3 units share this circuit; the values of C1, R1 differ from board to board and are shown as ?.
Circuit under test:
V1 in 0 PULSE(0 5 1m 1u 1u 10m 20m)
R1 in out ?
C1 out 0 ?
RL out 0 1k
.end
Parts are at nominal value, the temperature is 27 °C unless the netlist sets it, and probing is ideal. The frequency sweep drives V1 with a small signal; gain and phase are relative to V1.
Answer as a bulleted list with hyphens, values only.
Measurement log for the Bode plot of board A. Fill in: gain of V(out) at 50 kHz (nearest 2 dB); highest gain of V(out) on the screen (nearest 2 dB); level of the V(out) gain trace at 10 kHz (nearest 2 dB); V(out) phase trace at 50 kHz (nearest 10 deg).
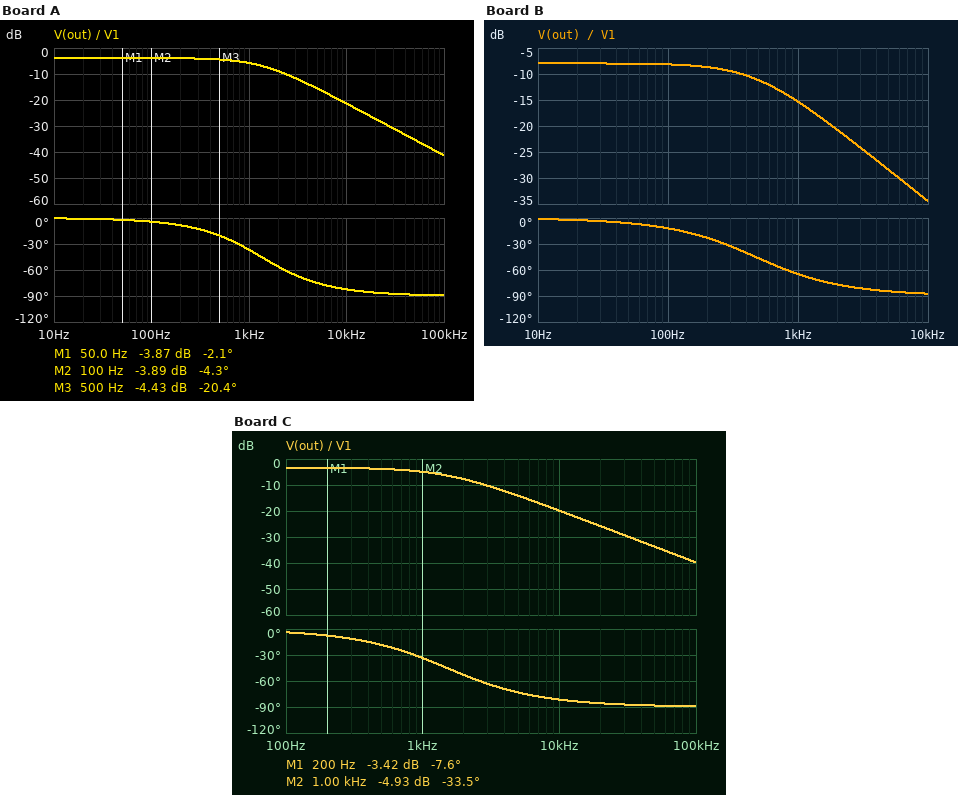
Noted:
- -36 dB
- -4 dB
- -22 dB
- -90 deg
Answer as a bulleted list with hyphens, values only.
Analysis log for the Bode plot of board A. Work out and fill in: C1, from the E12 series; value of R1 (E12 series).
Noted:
- 330 nF
- 560 Ω
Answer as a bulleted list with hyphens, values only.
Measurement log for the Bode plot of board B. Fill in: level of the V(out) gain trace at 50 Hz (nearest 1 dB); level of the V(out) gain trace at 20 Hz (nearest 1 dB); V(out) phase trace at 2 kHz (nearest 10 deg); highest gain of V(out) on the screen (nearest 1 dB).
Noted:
- -8 dB
- -8 dB
- -80 deg
- -8 dB
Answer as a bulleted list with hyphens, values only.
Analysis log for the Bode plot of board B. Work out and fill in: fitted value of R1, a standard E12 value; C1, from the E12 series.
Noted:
- 1.5 kΩ
- 560 nF
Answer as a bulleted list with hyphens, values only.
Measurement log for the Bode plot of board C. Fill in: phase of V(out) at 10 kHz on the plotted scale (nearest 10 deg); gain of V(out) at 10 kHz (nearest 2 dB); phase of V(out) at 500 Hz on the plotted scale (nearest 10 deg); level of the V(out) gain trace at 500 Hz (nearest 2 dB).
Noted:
- -80 deg
- -20 dB
- -20 deg
- -4 dB
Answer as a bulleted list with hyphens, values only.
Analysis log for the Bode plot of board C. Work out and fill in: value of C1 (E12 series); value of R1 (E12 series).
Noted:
- 330 nF
- 470 Ω
